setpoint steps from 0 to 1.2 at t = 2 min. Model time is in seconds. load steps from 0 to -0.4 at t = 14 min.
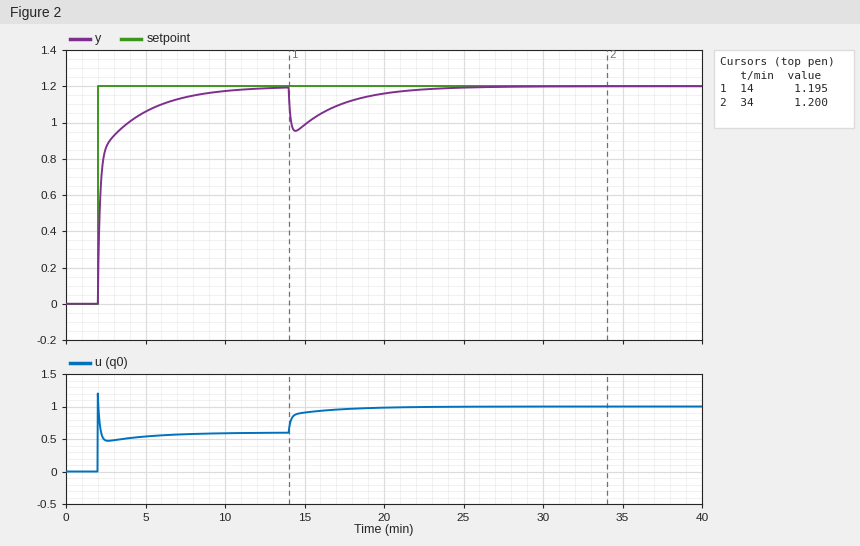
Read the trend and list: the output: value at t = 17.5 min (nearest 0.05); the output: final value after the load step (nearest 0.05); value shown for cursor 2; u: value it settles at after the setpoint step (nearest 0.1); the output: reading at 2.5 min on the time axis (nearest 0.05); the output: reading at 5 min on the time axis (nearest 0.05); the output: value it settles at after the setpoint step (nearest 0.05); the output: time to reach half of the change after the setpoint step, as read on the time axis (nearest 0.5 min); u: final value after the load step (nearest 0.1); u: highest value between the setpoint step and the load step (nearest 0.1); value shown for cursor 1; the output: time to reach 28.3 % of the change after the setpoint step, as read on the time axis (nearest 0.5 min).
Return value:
1.10
1.20
1.200
0.6
0.85
1.05
1.20
2.0 min
1.0
1.2
1.195
2.0 min
